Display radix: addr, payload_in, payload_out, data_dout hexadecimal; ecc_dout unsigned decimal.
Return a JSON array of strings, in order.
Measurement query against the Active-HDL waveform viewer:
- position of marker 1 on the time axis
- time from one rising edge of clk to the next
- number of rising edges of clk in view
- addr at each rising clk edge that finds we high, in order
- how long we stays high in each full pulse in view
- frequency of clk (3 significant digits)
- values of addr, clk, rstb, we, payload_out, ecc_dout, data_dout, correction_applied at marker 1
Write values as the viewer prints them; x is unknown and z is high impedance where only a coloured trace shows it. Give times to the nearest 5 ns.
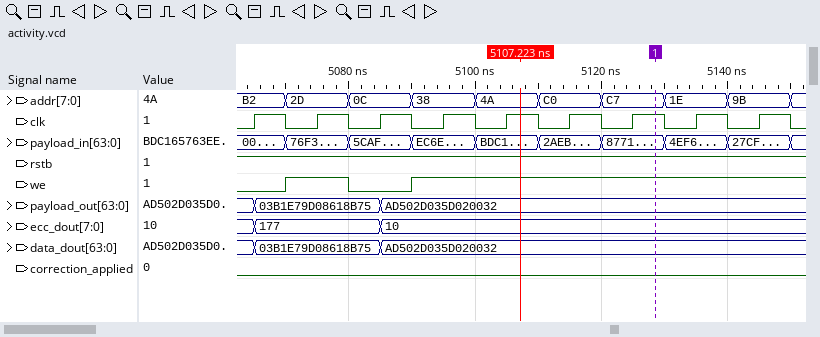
["5130 ns", "10 ns", "9", "2D, 38, 4A, C0, C7, 1E, 9B", "10 ns", "100 MHz", "addr=C7, clk=1, rstb=1, we=1, payload_out=AD502D035D020032, ecc_dout=10, data_dout=AD502D035D020032, correction_applied=0"]
